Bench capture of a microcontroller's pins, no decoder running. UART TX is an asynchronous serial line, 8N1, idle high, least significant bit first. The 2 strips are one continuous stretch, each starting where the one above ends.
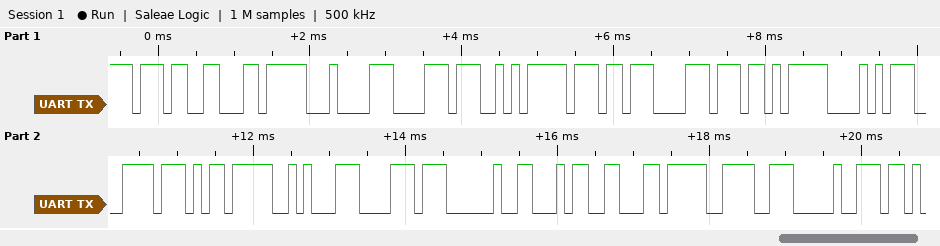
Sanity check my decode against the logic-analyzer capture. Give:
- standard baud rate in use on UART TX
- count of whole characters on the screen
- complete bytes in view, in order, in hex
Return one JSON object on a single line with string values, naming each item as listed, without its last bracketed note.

{"standard baud rate in use on UART TX": "9600 baud", "count of whole characters on the screen": "18", "complete bytes in view, in order, in hex": "0x37 0xEC 0x84 0xB8 0xEA 0xB7 0xB8 0xEB 0xA8 0xBC 0xED 0x8A 0xB8 0x20 0x34 0xEC 0x9E 0x90"}
